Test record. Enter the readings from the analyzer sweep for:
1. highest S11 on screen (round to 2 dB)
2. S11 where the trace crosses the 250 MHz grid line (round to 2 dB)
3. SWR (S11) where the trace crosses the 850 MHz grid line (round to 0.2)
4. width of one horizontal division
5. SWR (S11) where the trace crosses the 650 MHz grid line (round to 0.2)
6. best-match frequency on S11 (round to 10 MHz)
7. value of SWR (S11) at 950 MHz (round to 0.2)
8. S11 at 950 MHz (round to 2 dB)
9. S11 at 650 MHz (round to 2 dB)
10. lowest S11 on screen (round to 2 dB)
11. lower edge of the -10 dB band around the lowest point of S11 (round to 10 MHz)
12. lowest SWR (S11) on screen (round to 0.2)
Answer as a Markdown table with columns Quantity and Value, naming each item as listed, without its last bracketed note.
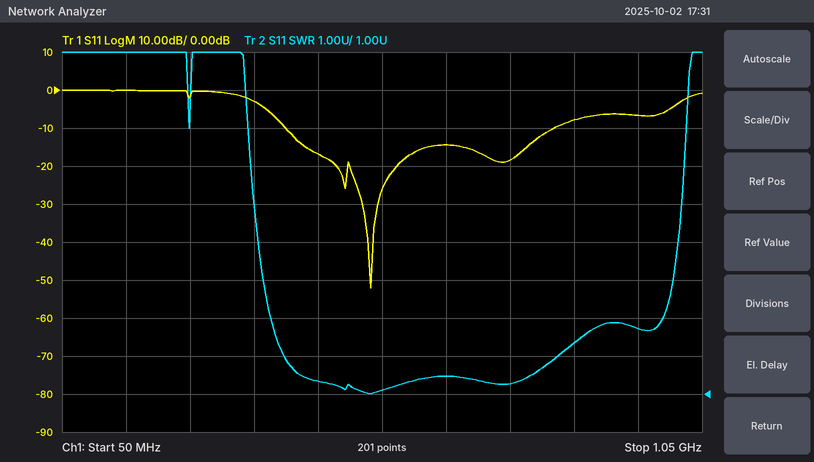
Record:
| Quantity | Value |
|---|---|
| highest S11 on screen | 0 dB |
| S11 where the trace crosses the 250 MHz grid line | -2 dB |
| SWR (S11) where the trace crosses the 850 MHz grid line | 2.4 |
| width of one horizontal division | 100 MHz |
| SWR (S11) where the trace crosses the 650 MHz grid line | 1.4 |
| best-match frequency on S11 | 530 MHz |
| value of SWR (S11) at 950 MHz | 2.8 |
| S11 at 950 MHz | -6 dB |
| S11 at 650 MHz | -14 dB |
| lowest S11 on screen | -52 dB |
| lower edge of the -10 dB band around the lowest point of S11 | 400 MHz |
| lowest SWR (S11) on screen | 1.0 |
